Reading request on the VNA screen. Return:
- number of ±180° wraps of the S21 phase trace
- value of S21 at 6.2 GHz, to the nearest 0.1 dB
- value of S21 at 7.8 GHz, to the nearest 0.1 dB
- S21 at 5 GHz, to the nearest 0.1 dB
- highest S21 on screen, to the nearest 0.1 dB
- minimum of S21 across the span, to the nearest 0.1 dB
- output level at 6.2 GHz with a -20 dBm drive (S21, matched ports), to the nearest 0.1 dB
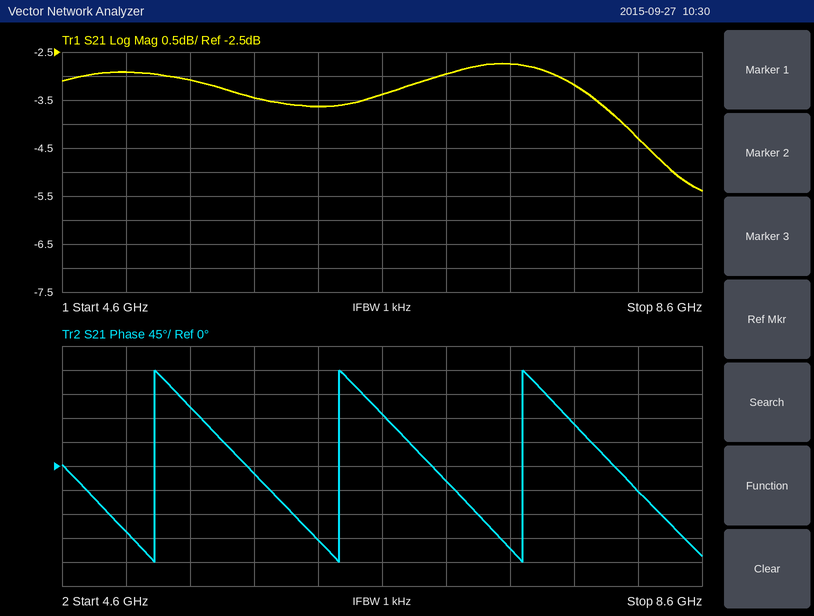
3
-3.6 dB
-3.2 dB
-2.9 dB
-2.7 dB
-5.4 dB
-23.6 dBm
